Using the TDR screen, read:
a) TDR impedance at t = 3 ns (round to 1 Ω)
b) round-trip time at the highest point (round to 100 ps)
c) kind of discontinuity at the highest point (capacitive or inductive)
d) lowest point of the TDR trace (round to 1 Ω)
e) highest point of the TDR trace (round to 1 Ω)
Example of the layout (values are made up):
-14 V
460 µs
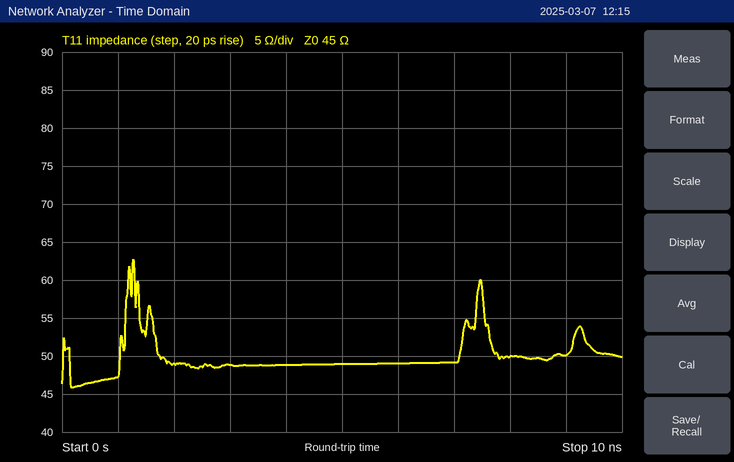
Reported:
49 Ω
1.3 ns
inductive
46 Ω
63 Ω
